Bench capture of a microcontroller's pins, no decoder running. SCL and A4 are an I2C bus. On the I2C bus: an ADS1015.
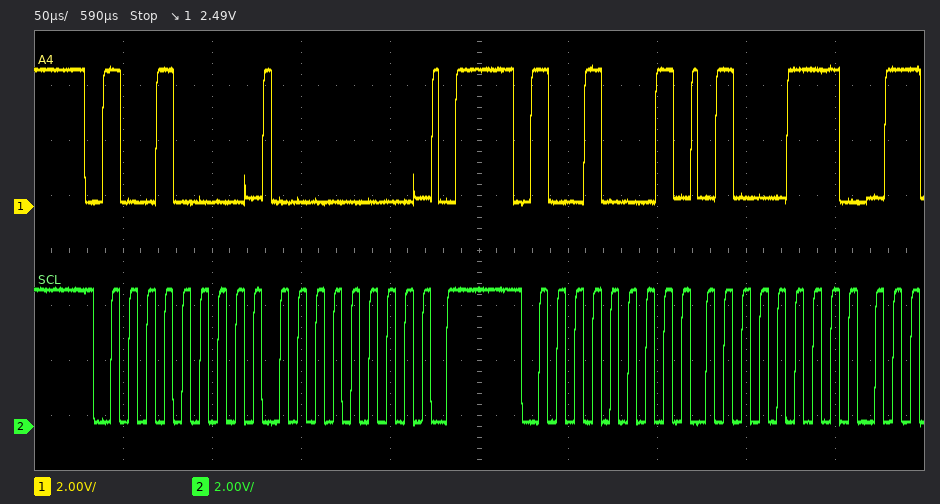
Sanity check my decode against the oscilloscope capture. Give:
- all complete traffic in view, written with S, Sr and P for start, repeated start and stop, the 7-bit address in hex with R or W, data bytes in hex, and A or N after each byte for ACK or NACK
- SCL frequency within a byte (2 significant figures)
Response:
S 48W A 00 A P S 48R A 47 A
100 kHz
